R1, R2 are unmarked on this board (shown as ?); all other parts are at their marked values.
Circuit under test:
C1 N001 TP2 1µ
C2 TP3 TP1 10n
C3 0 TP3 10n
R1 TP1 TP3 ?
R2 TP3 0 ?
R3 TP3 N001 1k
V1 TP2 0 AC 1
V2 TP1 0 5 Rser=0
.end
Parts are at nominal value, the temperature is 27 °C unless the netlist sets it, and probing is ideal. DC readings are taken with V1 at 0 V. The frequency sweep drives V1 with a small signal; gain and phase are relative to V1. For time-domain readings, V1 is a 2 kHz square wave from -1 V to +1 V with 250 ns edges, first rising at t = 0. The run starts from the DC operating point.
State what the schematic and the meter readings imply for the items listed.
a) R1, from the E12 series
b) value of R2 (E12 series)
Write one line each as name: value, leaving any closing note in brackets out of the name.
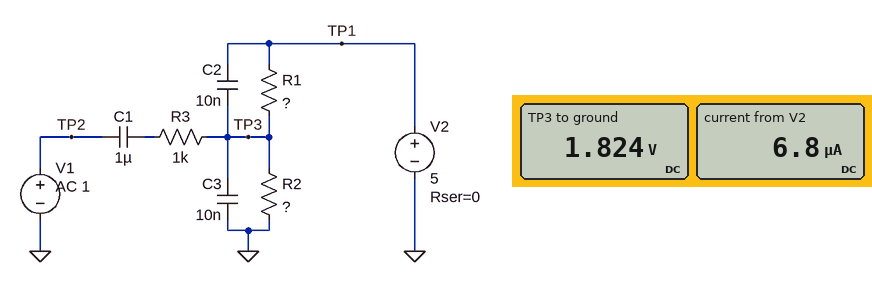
R1, from the E12 series: 470 kΩ
value of R2: 270 kΩ
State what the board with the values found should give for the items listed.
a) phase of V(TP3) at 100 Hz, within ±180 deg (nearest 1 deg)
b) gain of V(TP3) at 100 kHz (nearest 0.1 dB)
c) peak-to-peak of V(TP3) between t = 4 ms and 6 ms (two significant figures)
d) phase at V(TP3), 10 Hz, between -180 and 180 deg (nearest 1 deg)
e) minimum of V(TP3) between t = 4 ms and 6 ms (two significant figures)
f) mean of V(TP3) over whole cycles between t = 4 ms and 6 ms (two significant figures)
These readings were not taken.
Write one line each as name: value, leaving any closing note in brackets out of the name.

phase of V(TP3) at 100 Hz, within ±180 deg: 0 deg
gain of V(TP3) at 100 kHz: -22.0 dB
peak-to-peak of V(TP3) between t = 4 ms and 6 ms: 2.0 V
phase at V(TP3), 10 Hz, between -180 and 180 deg: 5 deg
minimum of V(TP3) between t = 4 ms and 6 ms: 1.8 V
mean of V(TP3) over whole cycles between t = 4 ms and 6 ms: 2.8 V
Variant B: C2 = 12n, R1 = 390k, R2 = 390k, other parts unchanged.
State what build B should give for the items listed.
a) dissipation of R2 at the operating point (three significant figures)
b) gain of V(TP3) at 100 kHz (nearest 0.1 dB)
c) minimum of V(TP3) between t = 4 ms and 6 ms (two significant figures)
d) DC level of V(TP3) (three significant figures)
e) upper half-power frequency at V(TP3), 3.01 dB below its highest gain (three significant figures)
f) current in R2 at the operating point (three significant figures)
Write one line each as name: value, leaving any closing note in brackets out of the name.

dissipation of R2 at the operating point: 16.0 µW
gain of V(TP3) at 100 kHz: -22.8 dB
minimum of V(TP3) between t = 4 ms and 6 ms: 2.5 V
DC level of V(TP3): 2.50 V
upper half-power frequency at V(TP3), 3.01 dB below its highest gain: 7.43 kHz
current in R2 at the operating point: 6.41 µA
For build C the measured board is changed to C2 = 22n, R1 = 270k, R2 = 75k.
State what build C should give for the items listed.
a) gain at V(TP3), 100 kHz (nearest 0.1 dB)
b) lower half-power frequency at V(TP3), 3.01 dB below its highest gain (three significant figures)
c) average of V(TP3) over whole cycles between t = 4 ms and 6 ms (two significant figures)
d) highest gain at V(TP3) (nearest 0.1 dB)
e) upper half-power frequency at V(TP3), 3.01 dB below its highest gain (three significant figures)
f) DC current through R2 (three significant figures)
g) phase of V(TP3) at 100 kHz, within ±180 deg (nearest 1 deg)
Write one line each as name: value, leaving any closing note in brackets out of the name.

gain at V(TP3), 100 kHz: -26.1 dB
lower half-power frequency at V(TP3), 3.01 dB below its highest gain: 2.58 Hz
average of V(TP3) over whole cycles between t = 4 ms and 6 ms: 2.0 V
highest gain at V(TP3): -0.4 dB
upper half-power frequency at V(TP3), 3.01 dB below its highest gain: 5.22 kHz
DC current through R2: 14.5 µA
phase of V(TP3) at 100 kHz, within ±180 deg: -87 deg
